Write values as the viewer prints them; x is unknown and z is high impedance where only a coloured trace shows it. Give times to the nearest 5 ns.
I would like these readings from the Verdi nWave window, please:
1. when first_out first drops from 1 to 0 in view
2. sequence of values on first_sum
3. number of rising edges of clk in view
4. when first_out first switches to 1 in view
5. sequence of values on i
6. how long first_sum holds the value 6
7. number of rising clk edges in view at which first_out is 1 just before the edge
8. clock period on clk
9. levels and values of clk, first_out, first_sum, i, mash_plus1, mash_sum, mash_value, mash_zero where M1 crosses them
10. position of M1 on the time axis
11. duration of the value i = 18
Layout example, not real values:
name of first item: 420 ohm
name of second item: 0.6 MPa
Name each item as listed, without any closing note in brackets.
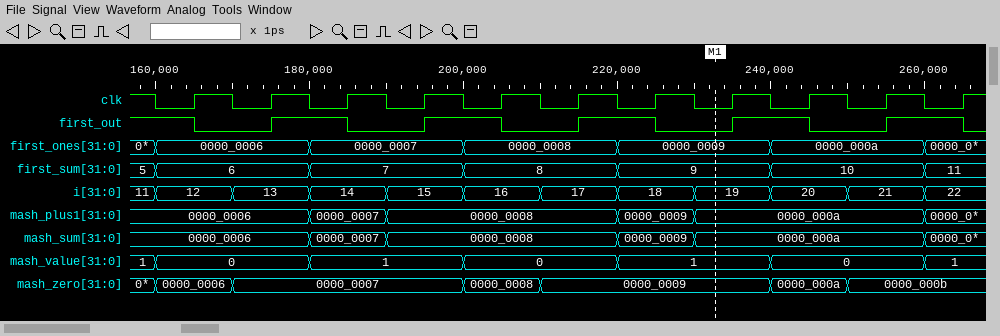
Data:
when first_out first drops from 1 to 0 in view: 165 ns
sequence of values on first_sum: 5, 6, 7, 8, 9, 10, 11
number of rising edges of clk in view: 11
when first_out first switches to 1 in view: 175 ns
sequence of values on i: 11, 12, 13, 14, 15, 16, 17, 18, 19, 20, 21, 22
how long first_sum holds the value 6: 20 ns
number of rising clk edges in view at which first_out is 1 just before the edge: 6
clock period on clk: 10 ns
levels and values of clk, first_out, first_sum, i, mash_plus1, mash_sum, mash_value, mash_zero where M1 crosses them: clk=0, first_out=0, first_sum=9, i=19, mash_plus1=0000_000a, mash_sum=0000_000a, mash_value=1, mash_zero=0000_0009
position of M1 on the time axis: 235 ns
duration of the value i = 18: 10 ns
